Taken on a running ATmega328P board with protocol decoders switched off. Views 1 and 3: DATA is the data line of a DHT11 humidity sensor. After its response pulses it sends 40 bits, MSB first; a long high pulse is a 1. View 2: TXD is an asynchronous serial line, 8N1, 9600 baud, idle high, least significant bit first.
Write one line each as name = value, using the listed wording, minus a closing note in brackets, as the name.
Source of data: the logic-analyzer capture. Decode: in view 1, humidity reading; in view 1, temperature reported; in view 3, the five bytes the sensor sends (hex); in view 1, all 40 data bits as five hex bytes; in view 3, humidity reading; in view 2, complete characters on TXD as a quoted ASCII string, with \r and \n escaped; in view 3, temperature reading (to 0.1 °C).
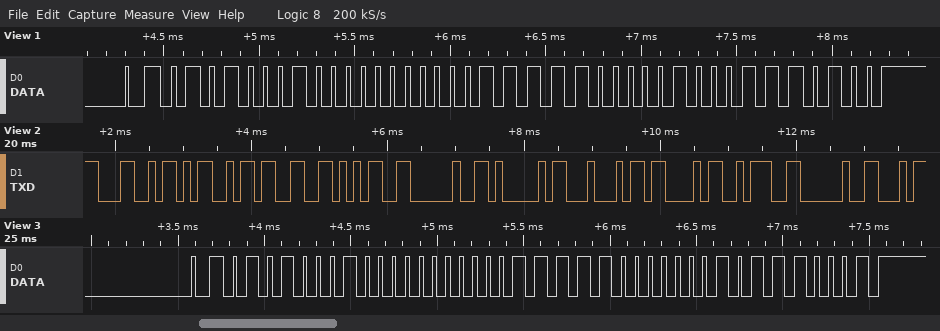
in view 1, humidity reading = 81 %
in view 1, temperature reported = 31.4 °C
in view 3, the five bytes the sensor sends = 51 00 1F 01 71
in view 1, all 40 data bits as five hex bytes = 51 00 1F 04 74
in view 3, humidity reading = 81 %
in view 2, complete characters on TXD as a quoted ASCII string, with \r and \n escaped = "LM35 ADC: "
in view 3, temperature reading = 31.1 °C
